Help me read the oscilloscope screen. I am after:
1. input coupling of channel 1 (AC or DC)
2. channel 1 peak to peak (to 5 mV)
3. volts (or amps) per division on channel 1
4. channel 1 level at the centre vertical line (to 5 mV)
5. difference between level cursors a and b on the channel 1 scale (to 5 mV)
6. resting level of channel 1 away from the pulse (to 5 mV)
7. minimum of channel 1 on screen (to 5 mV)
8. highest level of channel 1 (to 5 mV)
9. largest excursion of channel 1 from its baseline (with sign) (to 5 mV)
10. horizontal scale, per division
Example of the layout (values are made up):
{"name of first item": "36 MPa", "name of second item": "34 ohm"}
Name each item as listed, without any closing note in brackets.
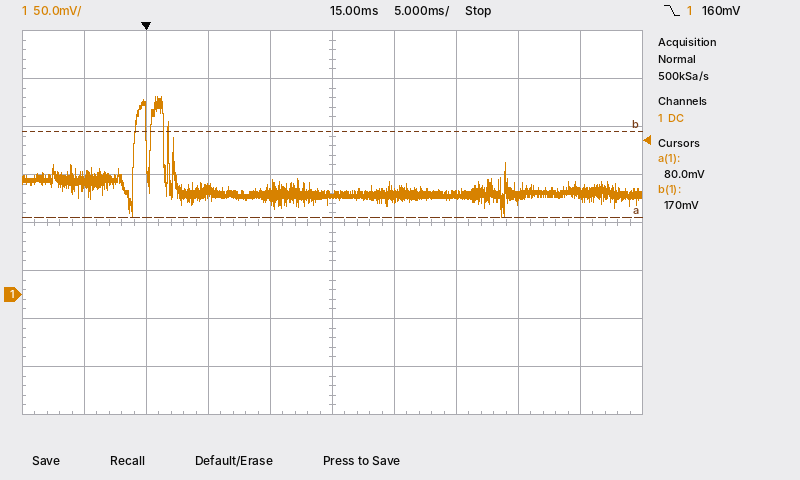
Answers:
{"input coupling of channel 1": "DC", "channel 1 peak to peak": "125 mV", "volts (or amps) per division on channel 1": "50 mV", "channel 1 level at the centre vertical line": "105 mV", "difference between level cursors a and b on the channel 1 scale": "90 mV", "resting level of channel 1 away from the pulse": "105 mV", "minimum of channel 1 on screen": "80 mV", "highest level of channel 1": "205 mV", "largest excursion of channel 1 from its baseline (with sign)": "+100 mV", "horizontal scale, per division": "5 ms"}
